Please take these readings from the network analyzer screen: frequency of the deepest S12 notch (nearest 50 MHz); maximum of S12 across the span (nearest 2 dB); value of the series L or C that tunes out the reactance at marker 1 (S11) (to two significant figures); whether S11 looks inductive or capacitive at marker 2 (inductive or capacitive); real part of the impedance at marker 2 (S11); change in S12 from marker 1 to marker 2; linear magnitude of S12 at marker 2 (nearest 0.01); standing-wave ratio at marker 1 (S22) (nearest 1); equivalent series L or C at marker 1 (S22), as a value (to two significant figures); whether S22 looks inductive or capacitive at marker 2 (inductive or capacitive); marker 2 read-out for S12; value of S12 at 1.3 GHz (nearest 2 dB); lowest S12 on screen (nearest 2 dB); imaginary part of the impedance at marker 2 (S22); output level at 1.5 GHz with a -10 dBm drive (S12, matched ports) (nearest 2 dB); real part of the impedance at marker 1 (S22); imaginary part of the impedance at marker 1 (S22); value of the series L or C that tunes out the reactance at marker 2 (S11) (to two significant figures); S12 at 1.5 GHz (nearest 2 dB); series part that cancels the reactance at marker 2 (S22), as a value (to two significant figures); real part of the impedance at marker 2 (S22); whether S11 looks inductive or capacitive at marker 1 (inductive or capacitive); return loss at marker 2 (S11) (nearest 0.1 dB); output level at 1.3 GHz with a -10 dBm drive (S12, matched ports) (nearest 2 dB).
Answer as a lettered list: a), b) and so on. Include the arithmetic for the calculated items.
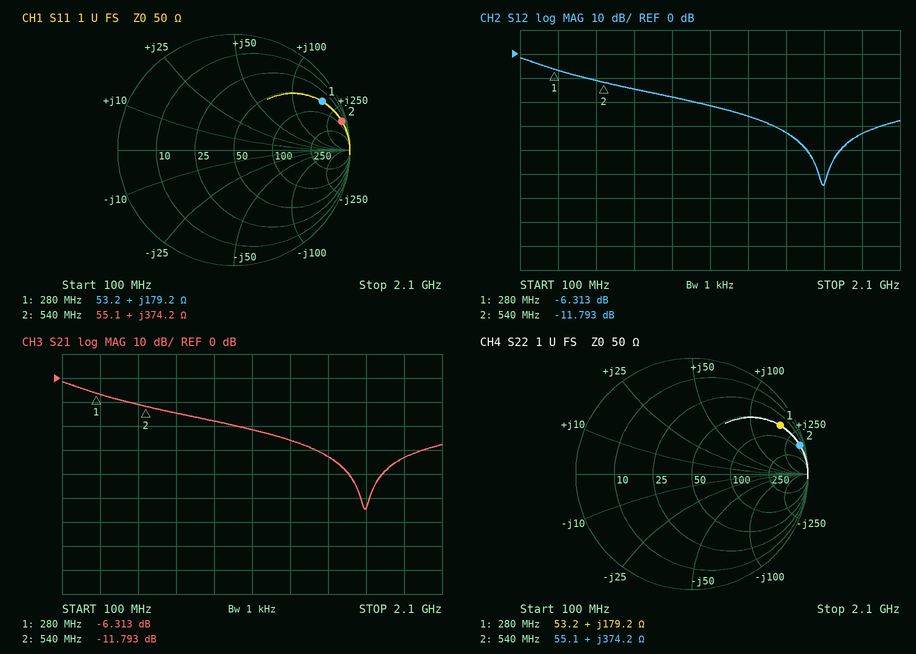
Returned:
a) 1.70 GHz
b) -2 dB
c) C = 1/(2π × 280 MHz × 179.2 Ω) ≈ 3.2 pF
d) inductive
e) 55.1 Ω
f) -11.793 − (-6.313) = -5.480 dB
g) 10^(-11.793/20) ≈ 0.26
h) 14
i) L = 179.2 Ω/(2π × 280 MHz) ≈ 102 nH, so 100 nH to two significant figures
j) inductive
k) -11.793 dB
l) -26 dB
m) -54 dB
n) +374.2 Ω
o) -10 dBm + (-32 dB) = -42 dBm
p) 53.2 Ω
q) +179.2 Ω
r) C = 1/(2π × 540 MHz × 374.2 Ω) ≈ 788 fF, so 790 fF to two significant figures
s) -32 dB
t) C = 1/(2π × 540 MHz × 374.2 Ω) ≈ 788 fF, so 790 fF to two significant figures
u) 55.1 Ω
v) inductive
w) 0.3 dB
x) -10 dBm + (-26 dB) = -36 dBm
